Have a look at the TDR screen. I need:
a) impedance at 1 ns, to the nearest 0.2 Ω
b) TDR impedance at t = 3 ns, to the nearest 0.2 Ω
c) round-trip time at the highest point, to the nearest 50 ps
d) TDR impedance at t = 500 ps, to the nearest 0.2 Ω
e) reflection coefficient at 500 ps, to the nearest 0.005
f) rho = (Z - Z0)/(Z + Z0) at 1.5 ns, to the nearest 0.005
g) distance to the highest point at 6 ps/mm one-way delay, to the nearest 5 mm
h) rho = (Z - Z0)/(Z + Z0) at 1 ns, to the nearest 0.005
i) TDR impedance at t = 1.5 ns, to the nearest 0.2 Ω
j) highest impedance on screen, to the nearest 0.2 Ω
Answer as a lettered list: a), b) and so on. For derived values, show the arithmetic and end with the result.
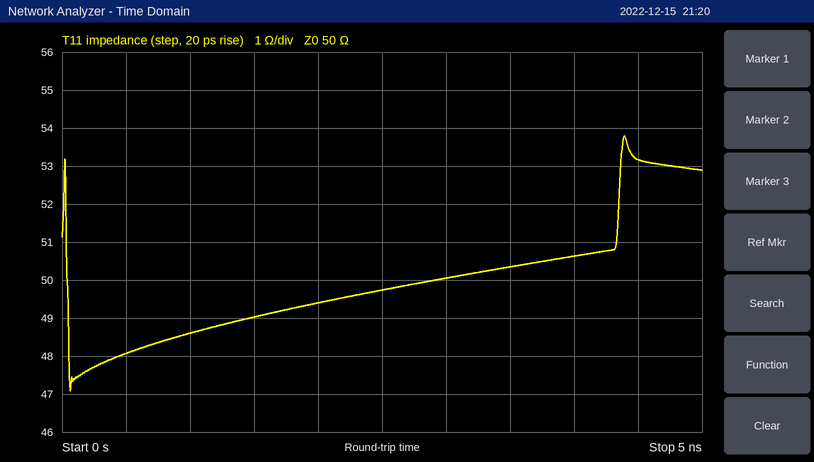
a) 48.6 Ω
b) 50.0 Ω
c) 4.40 ns
d) 48.0 Ω
e) (48 − 50)/(48 + 50) ≈ -0.020
f) (49 − 50)/(49 + 50) ≈ -0.010
g) 4.40 ns / 2 / 6 ps/mm ≈ 367 mm, so 365 mm to the nearest 5 mm
h) (48.6 − 50)/(48.6 + 50) ≈ -0.0142, so -0.015 to the nearest 0.005
i) 49.0 Ω
j) 53.8 Ω
